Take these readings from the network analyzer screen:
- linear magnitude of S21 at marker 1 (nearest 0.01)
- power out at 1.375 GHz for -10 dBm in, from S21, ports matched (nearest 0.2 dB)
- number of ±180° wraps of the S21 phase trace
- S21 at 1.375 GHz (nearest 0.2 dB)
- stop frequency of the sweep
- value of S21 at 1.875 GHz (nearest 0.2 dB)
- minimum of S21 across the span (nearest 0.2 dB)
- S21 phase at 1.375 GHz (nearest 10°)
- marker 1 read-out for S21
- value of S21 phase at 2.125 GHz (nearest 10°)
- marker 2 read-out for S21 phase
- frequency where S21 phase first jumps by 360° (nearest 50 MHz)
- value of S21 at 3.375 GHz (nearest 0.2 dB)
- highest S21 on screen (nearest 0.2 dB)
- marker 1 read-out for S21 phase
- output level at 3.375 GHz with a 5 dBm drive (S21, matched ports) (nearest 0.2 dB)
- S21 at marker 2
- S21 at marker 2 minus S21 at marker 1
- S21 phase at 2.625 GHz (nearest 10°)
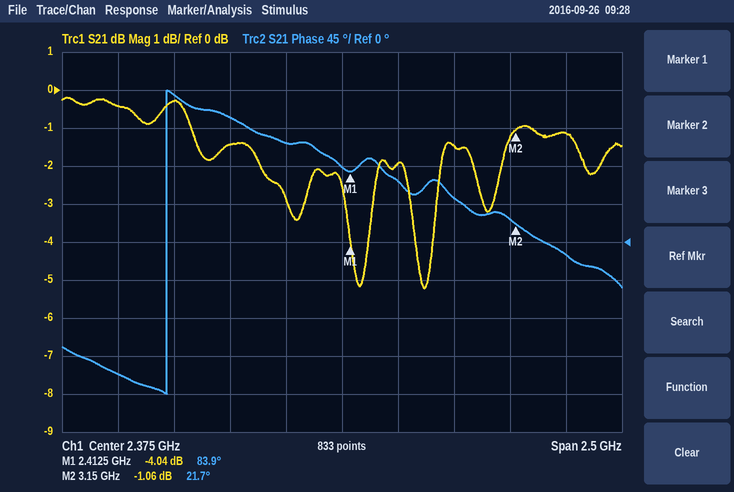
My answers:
0.63
-10.4 dBm
1
-0.4 dB
3.625 GHz
-1.4 dB
-5.2 dB
-160°
-4.04 dB
120°
21.7°
1.60 GHz
-1.2 dB
-0.2 dB
83.9°
3.8 dBm
-1.06 dB
2.98 dB
70°
